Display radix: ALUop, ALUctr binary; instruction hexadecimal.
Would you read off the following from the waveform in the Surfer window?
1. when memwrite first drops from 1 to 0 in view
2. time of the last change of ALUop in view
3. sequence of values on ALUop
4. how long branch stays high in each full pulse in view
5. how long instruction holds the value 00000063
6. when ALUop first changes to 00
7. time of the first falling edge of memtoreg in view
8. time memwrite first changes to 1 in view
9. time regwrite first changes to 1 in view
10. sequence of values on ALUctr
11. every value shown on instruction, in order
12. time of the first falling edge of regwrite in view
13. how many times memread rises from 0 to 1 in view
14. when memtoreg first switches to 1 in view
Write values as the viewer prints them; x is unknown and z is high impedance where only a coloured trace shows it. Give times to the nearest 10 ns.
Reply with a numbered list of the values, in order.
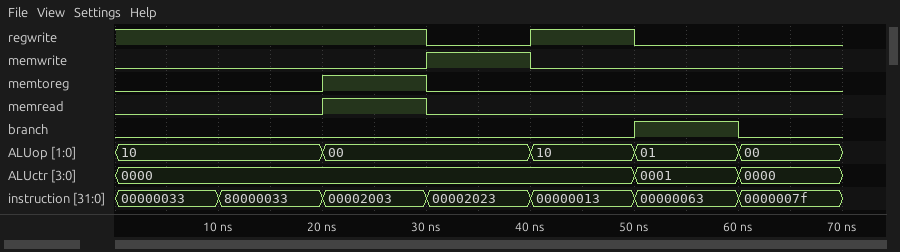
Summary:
1. 40 ns
2. 60 ns
3. 10, 00, 10, 01, 00
4. 10 ns
5. 10 ns
6. 20 ns
7. 30 ns
8. 30 ns
9. 40 ns
10. 0000, 0001, 0000
11. 00000033, 80000033, 00002003, 00002023, 00000013, 00000063, 0000007f
12. 30 ns
13. 1
14. 20 ns
